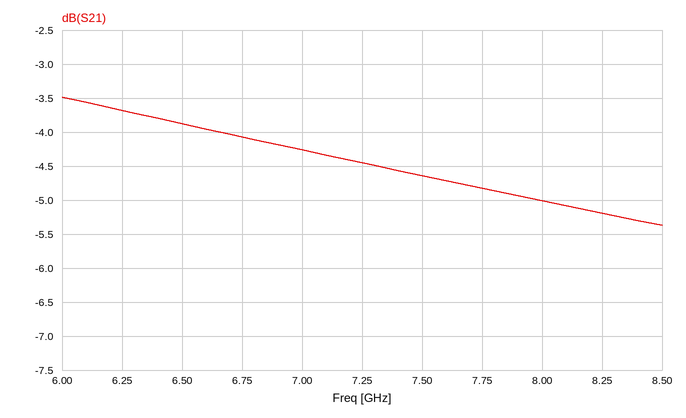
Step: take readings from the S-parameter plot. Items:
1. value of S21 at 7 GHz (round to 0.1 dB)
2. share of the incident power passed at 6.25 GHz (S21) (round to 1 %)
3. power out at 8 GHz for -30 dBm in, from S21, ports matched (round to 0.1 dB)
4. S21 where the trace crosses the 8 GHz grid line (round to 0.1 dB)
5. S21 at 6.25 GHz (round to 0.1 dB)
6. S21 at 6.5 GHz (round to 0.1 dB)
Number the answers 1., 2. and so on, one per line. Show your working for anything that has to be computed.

1. -4.3 dB
2. 10^(-3.7/10) ≈ 43 %
3. -30 dBm + (-5.0 dB) = -35.0 dBm
4. -5.0 dB
5. -3.7 dB
6. -3.9 dB
